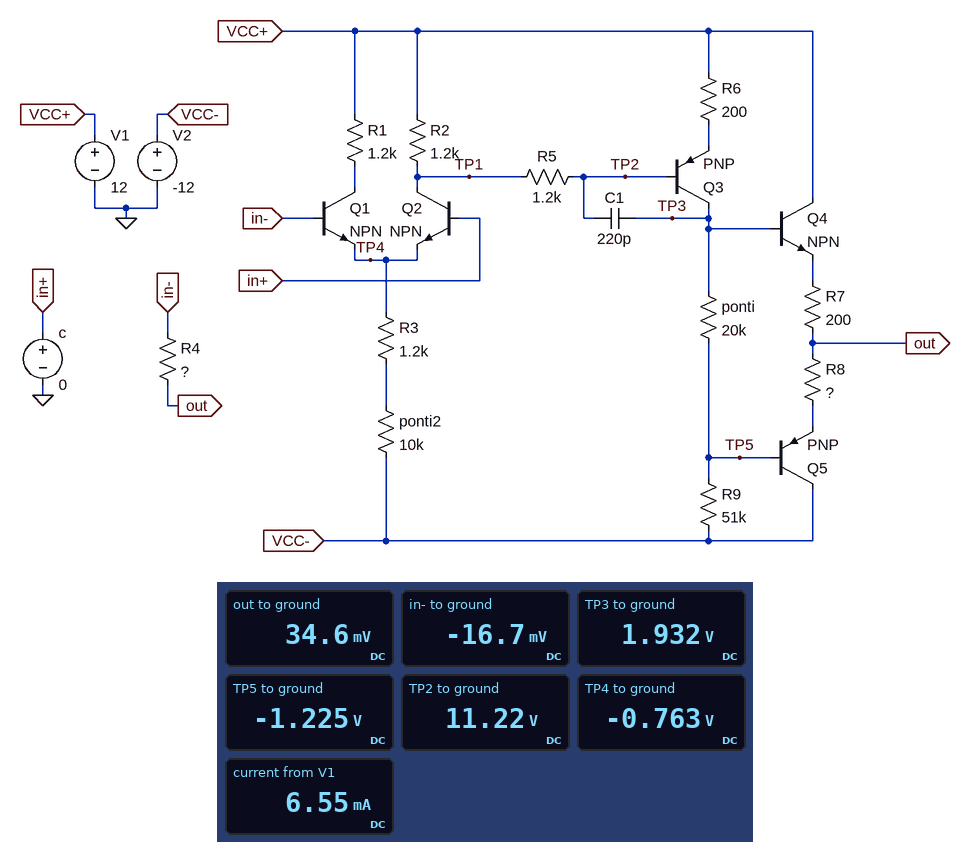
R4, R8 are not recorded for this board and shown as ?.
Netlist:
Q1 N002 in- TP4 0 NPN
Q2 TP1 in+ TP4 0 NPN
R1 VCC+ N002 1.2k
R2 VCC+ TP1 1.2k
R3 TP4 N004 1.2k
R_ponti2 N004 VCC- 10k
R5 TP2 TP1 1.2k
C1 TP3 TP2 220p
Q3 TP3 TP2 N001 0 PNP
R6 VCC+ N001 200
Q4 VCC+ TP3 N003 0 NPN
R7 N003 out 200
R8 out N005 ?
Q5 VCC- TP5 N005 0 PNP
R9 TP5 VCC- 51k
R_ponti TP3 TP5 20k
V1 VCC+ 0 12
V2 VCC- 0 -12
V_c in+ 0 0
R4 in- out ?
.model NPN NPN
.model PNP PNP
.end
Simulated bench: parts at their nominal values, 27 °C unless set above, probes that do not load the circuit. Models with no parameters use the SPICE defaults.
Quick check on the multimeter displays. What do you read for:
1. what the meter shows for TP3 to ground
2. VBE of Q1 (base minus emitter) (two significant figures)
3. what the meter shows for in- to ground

1.932 V
750 mV
-16.7 mV
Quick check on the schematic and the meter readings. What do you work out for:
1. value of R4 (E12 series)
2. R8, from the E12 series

15 kΩ
82 Ω
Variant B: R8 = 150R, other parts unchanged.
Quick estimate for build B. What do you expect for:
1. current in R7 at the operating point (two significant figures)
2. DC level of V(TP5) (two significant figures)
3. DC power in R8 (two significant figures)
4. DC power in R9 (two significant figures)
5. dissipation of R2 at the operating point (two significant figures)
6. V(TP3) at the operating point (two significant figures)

4.6 mA
-1.5 V
3.1 mW
2.2 mW
500 µW
1.8 V
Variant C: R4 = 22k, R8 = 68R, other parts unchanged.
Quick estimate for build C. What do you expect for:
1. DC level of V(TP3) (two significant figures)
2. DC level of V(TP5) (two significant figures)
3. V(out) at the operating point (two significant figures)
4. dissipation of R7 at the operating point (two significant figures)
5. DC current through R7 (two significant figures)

2.0 V
-1.1 V
58 mV
6.3 mW
5.6 mA
